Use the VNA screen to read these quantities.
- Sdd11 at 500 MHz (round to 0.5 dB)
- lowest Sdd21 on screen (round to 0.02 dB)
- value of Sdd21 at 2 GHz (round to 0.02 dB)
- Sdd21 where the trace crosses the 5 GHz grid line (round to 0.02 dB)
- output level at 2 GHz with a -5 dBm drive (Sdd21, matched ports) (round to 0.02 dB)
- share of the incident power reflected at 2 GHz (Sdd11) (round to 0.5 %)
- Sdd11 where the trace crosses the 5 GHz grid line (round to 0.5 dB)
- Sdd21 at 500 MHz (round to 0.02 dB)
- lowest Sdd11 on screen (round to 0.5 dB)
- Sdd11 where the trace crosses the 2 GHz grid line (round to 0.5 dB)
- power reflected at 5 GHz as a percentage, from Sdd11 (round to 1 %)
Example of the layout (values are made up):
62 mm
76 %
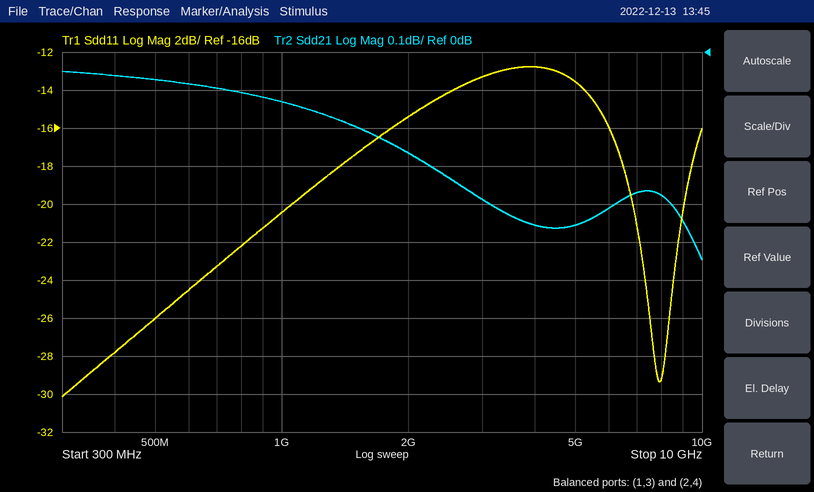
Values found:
-26.0 dB
-0.54 dB
-0.26 dB
-0.46 dB
-5.26 dBm
3.0 %
-13.5 dB
-0.08 dB
-30.0 dB
-15.5 dB
4 %
